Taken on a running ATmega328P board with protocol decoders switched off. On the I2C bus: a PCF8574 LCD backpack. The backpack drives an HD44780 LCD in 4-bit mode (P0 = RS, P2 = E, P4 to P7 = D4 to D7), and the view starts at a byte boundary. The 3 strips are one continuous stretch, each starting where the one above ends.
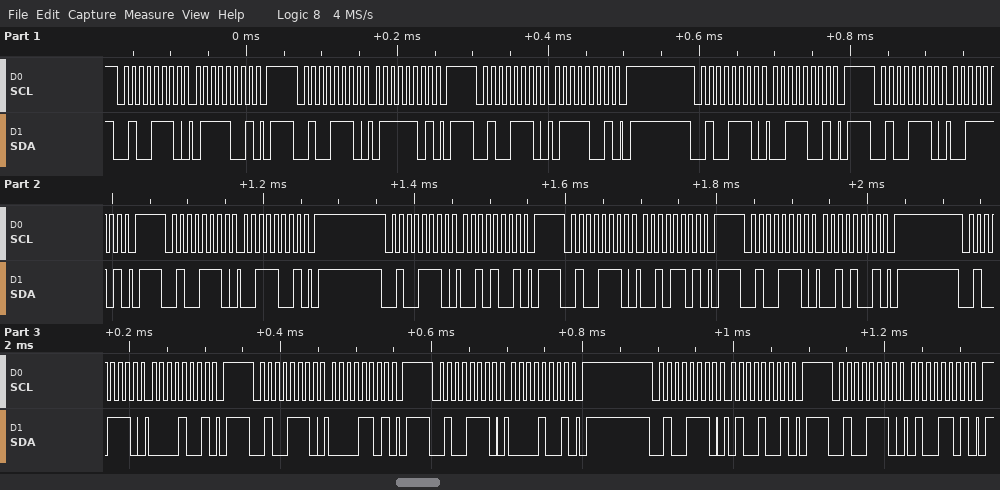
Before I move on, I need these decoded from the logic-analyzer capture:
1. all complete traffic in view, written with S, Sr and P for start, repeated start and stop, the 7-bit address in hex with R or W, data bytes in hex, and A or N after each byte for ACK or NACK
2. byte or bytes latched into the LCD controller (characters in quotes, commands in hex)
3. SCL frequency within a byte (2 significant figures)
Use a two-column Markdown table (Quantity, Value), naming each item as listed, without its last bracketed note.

| Quantity | Value |
|---|---|
| all complete traffic in view, written with S, Sr and P for start, repeated start and stop, the 7-bit address in hex with R or W, data bytes in hex, and A or N after each byte for ACK or NACK | S 27W A 79 A P S 27W A 7D A P S 27W A 79 A P S 27W A 39 A P S 27W A 3D A P S 27W A 39 A P S 27W A 29 A P S 27W A 2D A P S 27W A 29 A P S 27W A 09 A P S 27W A 0D A P S 27W A 09 A P S 27W A 49 A P S 27W A 4D A P |
| byte or bytes latched into the LCD controller | 's' ' ' |
| SCL frequency within a byte | 100 kHz |
